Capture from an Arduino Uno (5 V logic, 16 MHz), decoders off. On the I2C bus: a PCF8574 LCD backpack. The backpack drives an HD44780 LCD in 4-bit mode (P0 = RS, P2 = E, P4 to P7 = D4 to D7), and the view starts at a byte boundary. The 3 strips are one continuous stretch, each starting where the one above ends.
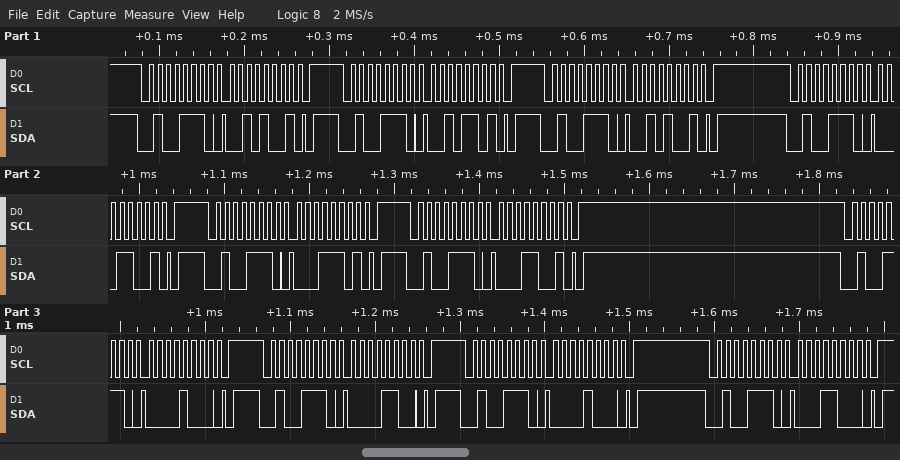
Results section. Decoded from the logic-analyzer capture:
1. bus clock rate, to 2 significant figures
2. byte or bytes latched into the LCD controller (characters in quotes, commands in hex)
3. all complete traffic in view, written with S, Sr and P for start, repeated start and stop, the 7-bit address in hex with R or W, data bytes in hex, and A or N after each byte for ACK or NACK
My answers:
100 kHz
'!'
S 27W A 29 A P S 27W A 2D A P S 27W A 29 A P S 27W A 19 A P S 27W A 1D A P S 27W A 19 A P S 27W A 08 A P S 27W A 0C A P S 27W A 08 A P S 27W A 18 A P
